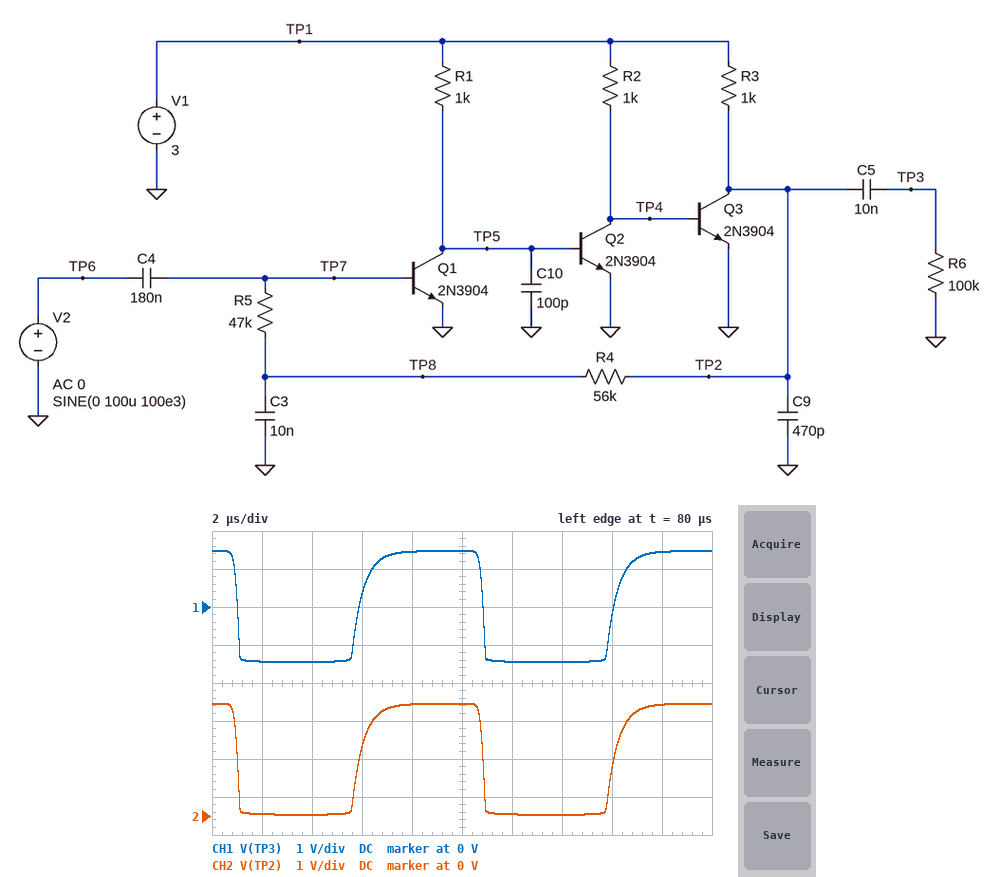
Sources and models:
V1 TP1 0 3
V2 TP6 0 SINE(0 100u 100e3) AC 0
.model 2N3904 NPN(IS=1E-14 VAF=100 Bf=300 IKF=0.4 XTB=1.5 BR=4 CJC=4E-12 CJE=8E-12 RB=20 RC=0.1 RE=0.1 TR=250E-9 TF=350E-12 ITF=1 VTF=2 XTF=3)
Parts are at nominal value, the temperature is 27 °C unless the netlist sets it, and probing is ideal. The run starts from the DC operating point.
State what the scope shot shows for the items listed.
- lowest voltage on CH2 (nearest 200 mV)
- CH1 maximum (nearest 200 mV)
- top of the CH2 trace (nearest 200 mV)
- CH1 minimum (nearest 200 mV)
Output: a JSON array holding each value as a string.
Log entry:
["0 V", "1.4 V", "3.0 V", "-1.4 V"]
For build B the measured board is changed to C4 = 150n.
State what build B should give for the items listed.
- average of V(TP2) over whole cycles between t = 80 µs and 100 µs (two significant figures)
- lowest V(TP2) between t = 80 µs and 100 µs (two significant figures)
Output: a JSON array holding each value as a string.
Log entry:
["1.4 V", "30 mV"]
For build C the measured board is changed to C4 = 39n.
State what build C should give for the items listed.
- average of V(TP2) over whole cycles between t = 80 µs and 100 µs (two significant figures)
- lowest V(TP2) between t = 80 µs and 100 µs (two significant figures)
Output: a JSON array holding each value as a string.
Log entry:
["2.0 V", "38 mV"]
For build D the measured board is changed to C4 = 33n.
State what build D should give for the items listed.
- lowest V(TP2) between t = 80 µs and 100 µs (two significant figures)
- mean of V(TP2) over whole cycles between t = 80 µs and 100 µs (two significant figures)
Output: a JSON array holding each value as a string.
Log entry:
["30 mV", "1.9 V"]
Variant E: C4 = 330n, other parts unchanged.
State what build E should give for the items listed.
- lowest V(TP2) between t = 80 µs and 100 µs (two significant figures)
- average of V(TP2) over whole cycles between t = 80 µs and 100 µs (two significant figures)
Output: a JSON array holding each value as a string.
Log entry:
["38 mV", "1.7 V"]
